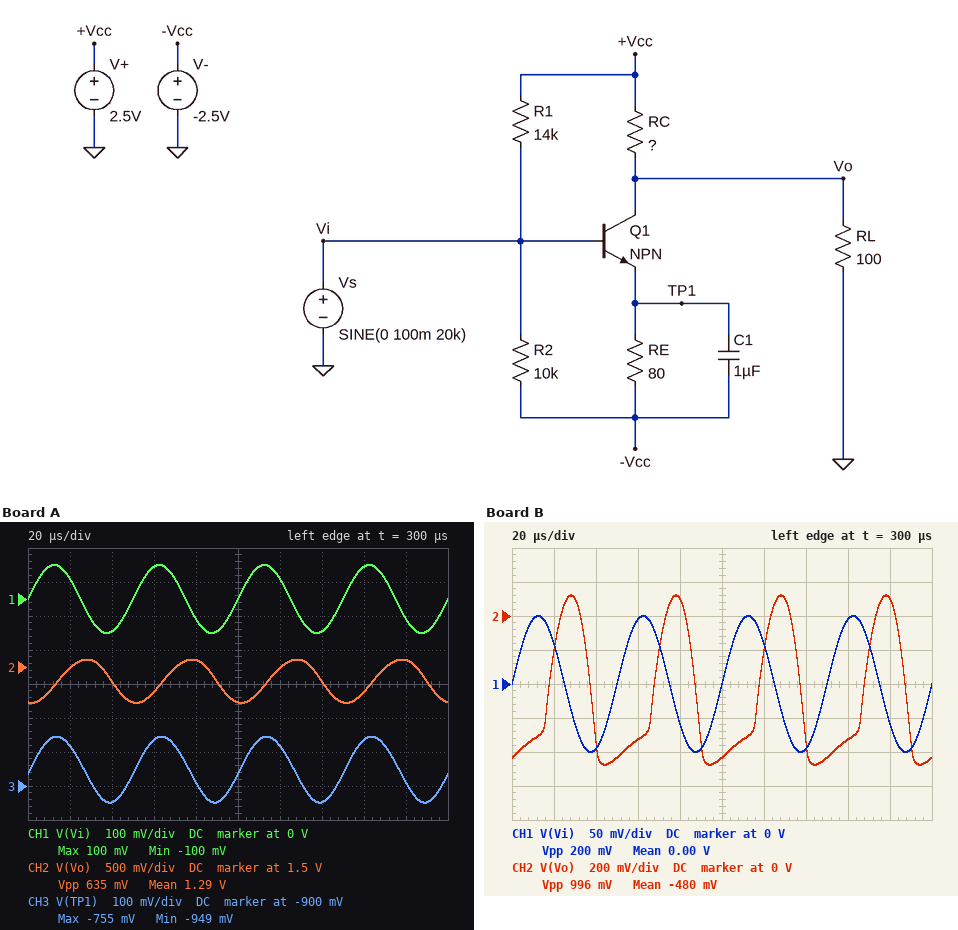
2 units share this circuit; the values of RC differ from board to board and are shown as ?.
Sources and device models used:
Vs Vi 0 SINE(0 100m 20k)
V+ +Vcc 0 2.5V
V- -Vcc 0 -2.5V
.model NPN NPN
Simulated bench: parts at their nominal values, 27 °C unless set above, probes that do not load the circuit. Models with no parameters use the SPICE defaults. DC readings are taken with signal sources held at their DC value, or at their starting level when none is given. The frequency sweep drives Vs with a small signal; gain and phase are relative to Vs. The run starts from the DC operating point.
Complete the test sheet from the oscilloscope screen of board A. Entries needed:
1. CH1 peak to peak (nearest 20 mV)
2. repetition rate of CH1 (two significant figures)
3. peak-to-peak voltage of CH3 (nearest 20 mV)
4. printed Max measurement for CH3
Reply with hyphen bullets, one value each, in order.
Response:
- 200 mV
- 20 kHz
- 200 mV
- -755 mV
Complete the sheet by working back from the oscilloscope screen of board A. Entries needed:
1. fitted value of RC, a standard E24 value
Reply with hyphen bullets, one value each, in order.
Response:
- 36 Ω
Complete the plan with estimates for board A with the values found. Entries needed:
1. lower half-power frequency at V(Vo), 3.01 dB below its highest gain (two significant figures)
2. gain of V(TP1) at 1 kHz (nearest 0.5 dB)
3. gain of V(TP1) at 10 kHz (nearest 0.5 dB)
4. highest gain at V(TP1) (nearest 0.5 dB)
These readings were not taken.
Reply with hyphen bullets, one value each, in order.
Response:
- 130 kHz
- 0 dB
- 0 dB
- 0 dB
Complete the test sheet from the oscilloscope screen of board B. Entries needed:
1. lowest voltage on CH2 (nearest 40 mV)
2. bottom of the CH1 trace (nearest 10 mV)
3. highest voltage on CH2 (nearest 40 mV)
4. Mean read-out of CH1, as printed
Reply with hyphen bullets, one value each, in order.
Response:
- -880 mV
- -100 mV
- 120 mV
- 0.00 V
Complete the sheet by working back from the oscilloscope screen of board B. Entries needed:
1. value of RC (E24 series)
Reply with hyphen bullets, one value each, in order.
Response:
- 240 Ω
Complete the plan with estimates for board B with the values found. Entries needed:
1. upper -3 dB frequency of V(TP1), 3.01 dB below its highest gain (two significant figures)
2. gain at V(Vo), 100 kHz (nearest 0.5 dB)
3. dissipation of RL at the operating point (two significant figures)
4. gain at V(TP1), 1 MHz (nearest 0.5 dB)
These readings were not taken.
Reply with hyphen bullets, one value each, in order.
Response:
- 110 kHz
- 29.0 dB
- 4.9 mW
- -19.0 dB
